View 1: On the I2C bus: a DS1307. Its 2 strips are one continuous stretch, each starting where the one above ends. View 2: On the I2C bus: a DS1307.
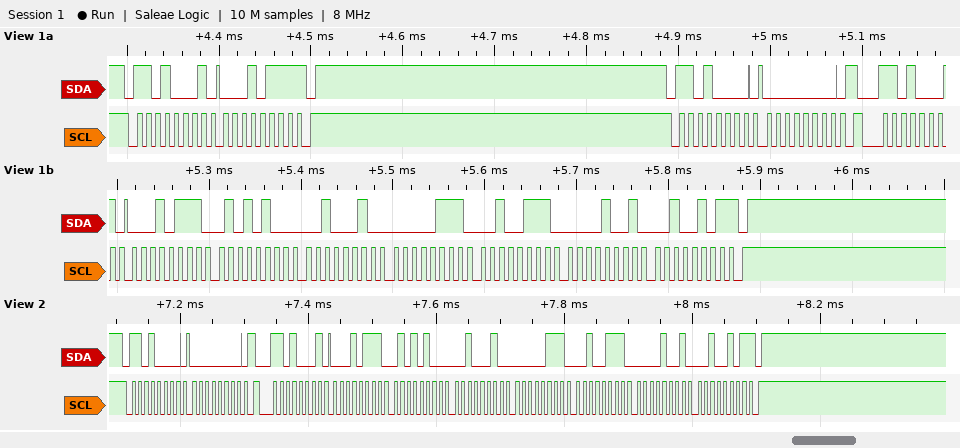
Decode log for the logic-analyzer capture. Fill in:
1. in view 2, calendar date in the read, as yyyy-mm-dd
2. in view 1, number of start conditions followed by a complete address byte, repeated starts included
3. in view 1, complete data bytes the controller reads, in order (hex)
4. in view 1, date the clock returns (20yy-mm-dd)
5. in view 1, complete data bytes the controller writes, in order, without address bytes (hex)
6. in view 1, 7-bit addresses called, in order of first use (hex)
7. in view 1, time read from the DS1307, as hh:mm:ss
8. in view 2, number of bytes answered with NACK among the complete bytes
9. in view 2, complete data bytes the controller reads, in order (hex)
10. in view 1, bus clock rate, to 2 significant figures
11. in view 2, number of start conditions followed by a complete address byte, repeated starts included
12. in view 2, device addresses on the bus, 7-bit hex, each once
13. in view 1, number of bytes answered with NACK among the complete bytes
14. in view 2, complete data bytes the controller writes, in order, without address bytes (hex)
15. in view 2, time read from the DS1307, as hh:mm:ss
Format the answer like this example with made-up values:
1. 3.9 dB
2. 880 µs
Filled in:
1. 2025-09-27
2. 3
3. 17 17 54 22 07 27 09 25
4. 2025-09-27
5. 00
6. 0x68
7. 22:54:17
8. 1
9. 17 54 22 07 27 09 25
10. 100 kHz
11. 2
12. 0x68
13. 2
14. 00
15. 22:54:17
